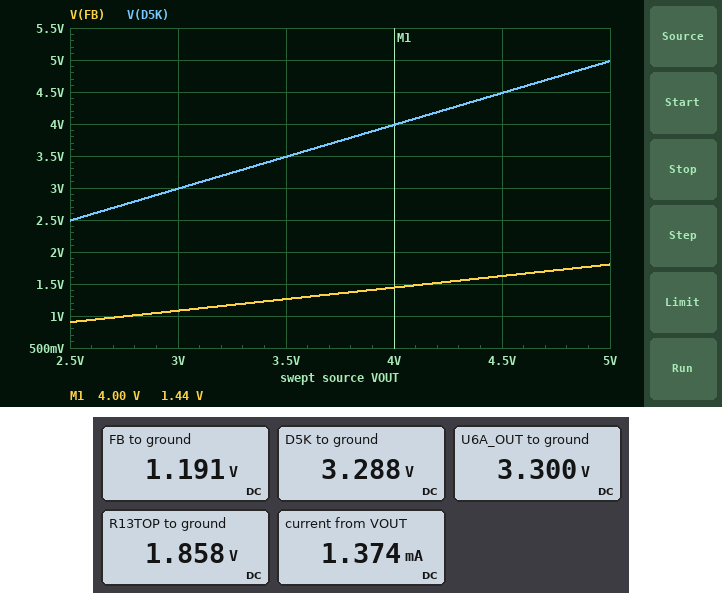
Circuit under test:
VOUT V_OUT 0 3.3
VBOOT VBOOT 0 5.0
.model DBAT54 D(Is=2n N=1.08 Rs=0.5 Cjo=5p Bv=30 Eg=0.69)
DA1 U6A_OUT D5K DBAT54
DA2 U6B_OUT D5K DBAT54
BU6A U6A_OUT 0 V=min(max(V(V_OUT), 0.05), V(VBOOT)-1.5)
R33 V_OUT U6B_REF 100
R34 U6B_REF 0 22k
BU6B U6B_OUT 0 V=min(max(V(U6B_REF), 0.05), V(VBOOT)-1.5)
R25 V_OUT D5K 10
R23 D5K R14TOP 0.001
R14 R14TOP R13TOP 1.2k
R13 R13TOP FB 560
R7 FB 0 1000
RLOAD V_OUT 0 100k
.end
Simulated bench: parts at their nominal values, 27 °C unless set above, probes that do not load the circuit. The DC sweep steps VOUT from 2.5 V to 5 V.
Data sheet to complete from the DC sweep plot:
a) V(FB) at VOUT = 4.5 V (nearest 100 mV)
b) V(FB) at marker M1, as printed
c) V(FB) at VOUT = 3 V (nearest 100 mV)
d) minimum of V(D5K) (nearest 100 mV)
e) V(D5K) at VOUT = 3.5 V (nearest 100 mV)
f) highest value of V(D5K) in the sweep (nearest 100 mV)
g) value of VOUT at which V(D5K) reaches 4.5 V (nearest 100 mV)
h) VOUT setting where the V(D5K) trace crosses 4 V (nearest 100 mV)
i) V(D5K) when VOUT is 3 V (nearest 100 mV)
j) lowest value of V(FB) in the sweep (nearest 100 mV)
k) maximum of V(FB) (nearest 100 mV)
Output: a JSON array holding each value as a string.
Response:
["1.6 V", "1.44 V", "1.1 V", "2.5 V", "3.5 V", "5.0 V", "4.5 V", "4.0 V", "3.0 V", "900 mV", "1.8 V"]
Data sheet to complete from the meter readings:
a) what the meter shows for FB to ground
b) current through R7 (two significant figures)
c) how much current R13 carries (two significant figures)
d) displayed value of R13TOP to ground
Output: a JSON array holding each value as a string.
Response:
["1.191 V", "1.2 mA", "1.2 mA", "1.858 V"]
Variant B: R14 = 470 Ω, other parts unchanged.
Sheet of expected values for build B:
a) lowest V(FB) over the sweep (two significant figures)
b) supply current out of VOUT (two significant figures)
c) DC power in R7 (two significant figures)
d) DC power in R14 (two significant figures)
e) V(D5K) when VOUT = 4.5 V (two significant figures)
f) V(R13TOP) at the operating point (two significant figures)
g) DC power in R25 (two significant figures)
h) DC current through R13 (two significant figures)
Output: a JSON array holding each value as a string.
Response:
["1.2 V", "1.8 mA", "2.6 mW", "1.2 mW", "4.5 V", "2.5 V", "26 µW", "1.6 mA"]
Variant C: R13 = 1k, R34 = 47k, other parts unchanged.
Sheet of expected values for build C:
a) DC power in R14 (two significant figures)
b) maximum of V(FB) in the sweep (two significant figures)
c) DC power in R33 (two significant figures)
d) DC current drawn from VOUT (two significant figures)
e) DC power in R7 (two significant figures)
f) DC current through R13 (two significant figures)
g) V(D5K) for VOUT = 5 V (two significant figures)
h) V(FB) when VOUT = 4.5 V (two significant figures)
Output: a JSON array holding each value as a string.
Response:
["1.3 mW", "1.6 V", "490 nW", "1.1 mA", "1.1 mW", "1.0 mA", "5.0 V", "1.4 V"]
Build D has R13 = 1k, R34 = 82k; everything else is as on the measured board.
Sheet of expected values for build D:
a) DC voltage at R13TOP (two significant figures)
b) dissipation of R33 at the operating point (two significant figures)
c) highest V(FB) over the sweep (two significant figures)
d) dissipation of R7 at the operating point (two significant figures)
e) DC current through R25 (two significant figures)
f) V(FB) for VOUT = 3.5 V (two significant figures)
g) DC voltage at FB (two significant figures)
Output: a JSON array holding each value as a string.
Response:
["2.1 V", "160 nW", "1.6 V", "1.1 mW", "1.0 mA", "1.1 V", "1.0 V"]
